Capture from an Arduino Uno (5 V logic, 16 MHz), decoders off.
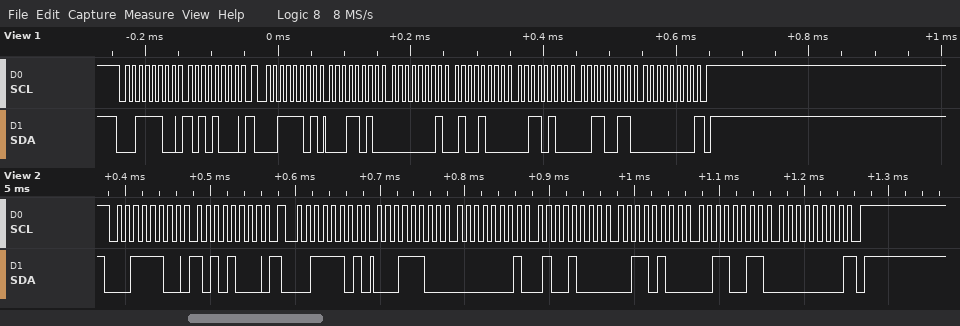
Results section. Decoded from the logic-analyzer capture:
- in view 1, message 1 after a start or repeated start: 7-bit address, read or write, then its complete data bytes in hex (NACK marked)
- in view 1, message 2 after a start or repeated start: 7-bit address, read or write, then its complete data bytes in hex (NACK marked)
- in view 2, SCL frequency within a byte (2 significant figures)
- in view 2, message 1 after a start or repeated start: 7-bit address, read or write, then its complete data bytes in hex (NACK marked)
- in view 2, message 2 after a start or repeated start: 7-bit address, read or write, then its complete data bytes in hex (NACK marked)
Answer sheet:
0x1E write: A8
0x1E read: 1A 01 48 34 33 00 NACK
100 kHz
0x1E write: A8
0x1E read: 1C 01 48 34 33 00 NACK
